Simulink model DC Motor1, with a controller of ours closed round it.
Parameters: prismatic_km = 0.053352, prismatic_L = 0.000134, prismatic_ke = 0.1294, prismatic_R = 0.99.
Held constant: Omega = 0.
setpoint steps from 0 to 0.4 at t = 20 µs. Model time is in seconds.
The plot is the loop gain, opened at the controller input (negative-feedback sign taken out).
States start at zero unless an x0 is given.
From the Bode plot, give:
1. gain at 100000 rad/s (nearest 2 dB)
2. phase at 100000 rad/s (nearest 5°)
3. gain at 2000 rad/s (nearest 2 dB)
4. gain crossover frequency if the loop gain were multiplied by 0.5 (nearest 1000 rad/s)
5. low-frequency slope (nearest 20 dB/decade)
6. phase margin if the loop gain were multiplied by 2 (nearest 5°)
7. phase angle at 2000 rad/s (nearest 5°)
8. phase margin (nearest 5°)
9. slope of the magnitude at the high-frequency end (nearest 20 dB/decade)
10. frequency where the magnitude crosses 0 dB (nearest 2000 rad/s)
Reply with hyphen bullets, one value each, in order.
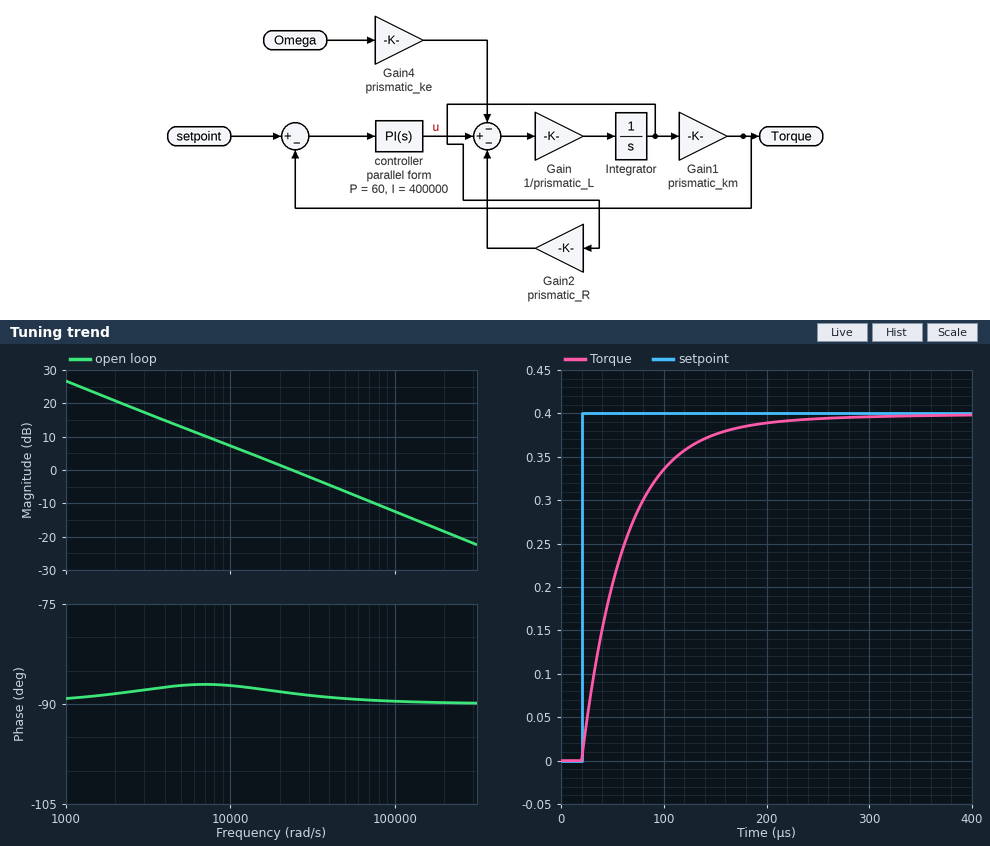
- -12 dB
- -90°
- 20 dB
- 12000 rad/s
- -20 dB/decade
- 90°
- -90°
- 90°
- -20 dB/decade
- 24000 rad/s
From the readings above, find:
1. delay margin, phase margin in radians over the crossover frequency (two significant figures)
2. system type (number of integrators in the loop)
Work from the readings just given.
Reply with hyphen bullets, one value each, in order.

- 0.000065 s
- 1
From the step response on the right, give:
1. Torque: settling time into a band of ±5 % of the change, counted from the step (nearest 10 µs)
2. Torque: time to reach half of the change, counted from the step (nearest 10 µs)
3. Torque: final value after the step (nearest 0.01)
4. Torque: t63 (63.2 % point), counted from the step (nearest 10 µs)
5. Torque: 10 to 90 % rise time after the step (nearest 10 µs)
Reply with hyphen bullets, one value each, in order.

- 140 µs
- 30 µs
- 0.40
- 40 µs
- 100 µs
